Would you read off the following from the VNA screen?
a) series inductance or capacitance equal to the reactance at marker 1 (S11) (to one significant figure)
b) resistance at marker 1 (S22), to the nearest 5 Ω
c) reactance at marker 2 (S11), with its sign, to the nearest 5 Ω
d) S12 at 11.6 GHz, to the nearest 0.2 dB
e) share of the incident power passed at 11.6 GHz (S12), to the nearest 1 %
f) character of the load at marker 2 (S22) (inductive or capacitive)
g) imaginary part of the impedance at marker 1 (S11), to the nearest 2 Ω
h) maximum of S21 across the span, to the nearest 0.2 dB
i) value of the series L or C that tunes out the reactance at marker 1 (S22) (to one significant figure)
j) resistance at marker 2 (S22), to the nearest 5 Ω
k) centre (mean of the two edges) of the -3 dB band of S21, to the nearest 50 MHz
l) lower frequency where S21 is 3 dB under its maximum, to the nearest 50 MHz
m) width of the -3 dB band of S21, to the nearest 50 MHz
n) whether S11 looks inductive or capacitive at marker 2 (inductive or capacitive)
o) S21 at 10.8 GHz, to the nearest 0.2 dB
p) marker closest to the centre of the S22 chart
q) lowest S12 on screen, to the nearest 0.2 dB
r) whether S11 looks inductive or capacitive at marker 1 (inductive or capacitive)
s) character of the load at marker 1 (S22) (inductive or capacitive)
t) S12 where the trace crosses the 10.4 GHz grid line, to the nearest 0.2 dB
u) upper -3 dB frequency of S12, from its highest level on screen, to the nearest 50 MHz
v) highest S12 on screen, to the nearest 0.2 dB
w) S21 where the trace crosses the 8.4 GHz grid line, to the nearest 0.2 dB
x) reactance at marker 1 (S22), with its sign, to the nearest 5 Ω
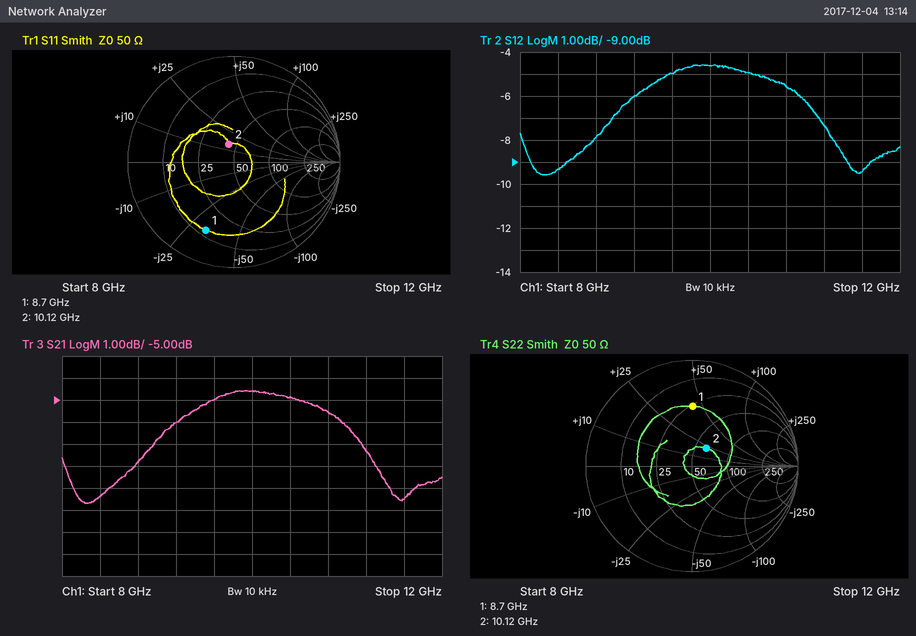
600 fF
25 Ω
+15 Ω
-9.4 dB
11 %
inductive
-32 Ω
-4.6 dB
400 fF
60 Ω
10.05 GHz
8.85 GHz
2.40 GHz
inductive
-5.6 dB
marker 2
-9.6 dB
capacitive
inductive
-5.0 dB
11.25 GHz
-4.6 dB
-9.4 dB
+45 Ω
